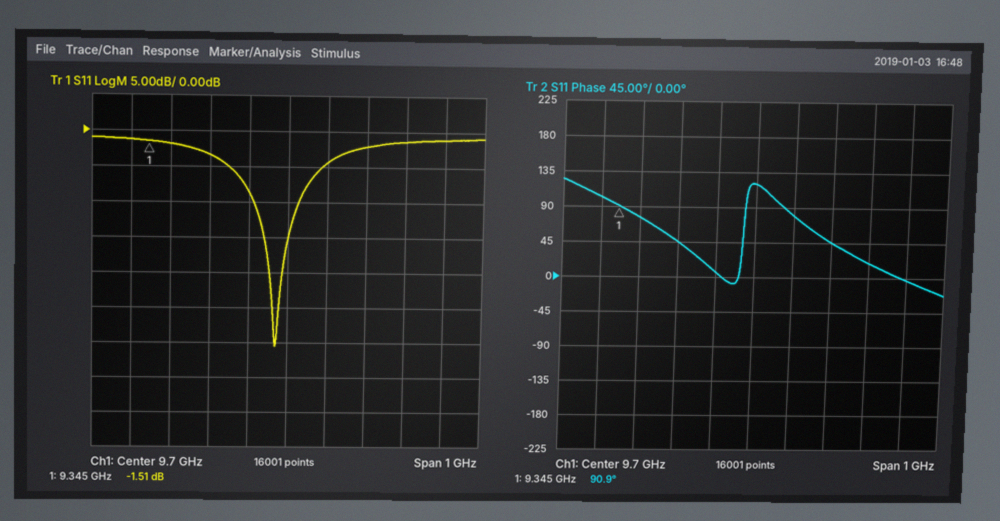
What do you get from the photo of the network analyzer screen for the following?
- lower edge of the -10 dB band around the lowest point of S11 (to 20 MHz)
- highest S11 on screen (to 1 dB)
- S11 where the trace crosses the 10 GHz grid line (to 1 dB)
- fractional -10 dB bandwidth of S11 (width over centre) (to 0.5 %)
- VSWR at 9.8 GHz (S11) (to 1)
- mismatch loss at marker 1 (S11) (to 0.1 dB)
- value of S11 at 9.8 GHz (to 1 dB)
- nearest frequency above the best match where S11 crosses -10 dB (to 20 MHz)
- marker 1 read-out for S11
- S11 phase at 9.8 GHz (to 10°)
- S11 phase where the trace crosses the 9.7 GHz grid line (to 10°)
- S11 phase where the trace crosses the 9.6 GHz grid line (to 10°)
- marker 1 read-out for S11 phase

9.62 GHz
-1 dB
-1 dB
1.0 %
4
5.3 dB
-4 dB
9.72 GHz
-1.51 dB
80°
120°
10°
90.9°
